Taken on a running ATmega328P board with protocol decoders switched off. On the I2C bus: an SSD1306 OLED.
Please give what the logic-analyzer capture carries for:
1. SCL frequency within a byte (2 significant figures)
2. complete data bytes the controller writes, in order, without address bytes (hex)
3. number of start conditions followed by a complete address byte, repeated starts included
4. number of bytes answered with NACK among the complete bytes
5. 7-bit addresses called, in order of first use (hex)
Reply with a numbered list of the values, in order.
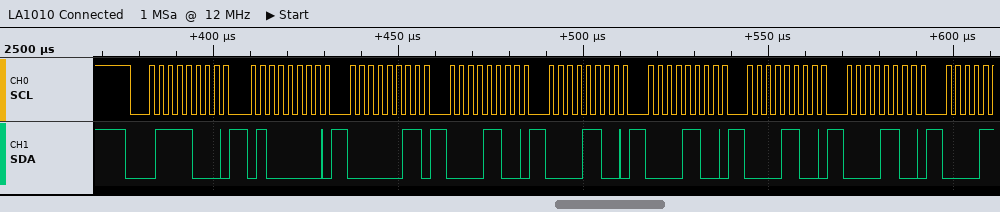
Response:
1. 400 kHz
2. 40 03 0C 0C 0C 0C 0C
3. 1
4. 0
5. 0x3C
